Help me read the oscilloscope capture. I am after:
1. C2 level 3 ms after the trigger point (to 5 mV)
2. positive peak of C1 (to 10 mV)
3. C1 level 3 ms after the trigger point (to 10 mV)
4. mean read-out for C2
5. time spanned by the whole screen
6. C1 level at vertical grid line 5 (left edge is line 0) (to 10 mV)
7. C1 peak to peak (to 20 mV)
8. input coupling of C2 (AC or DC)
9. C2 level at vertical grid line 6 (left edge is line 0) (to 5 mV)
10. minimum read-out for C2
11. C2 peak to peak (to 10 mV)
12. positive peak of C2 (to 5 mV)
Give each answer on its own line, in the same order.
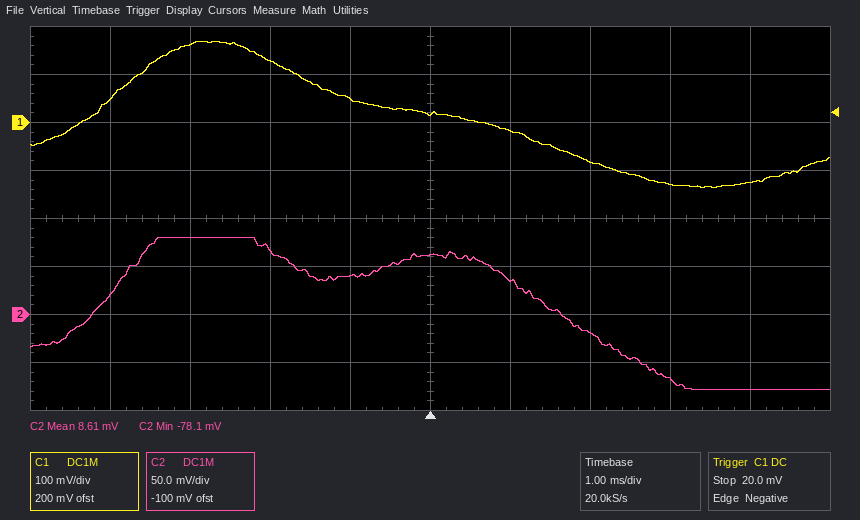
-70 mV
170 mV
-130 mV
8.61 mV
10 ms
20 mV
300 mV
DC
35 mV
-78.1 mV
160 mV
80 mV
